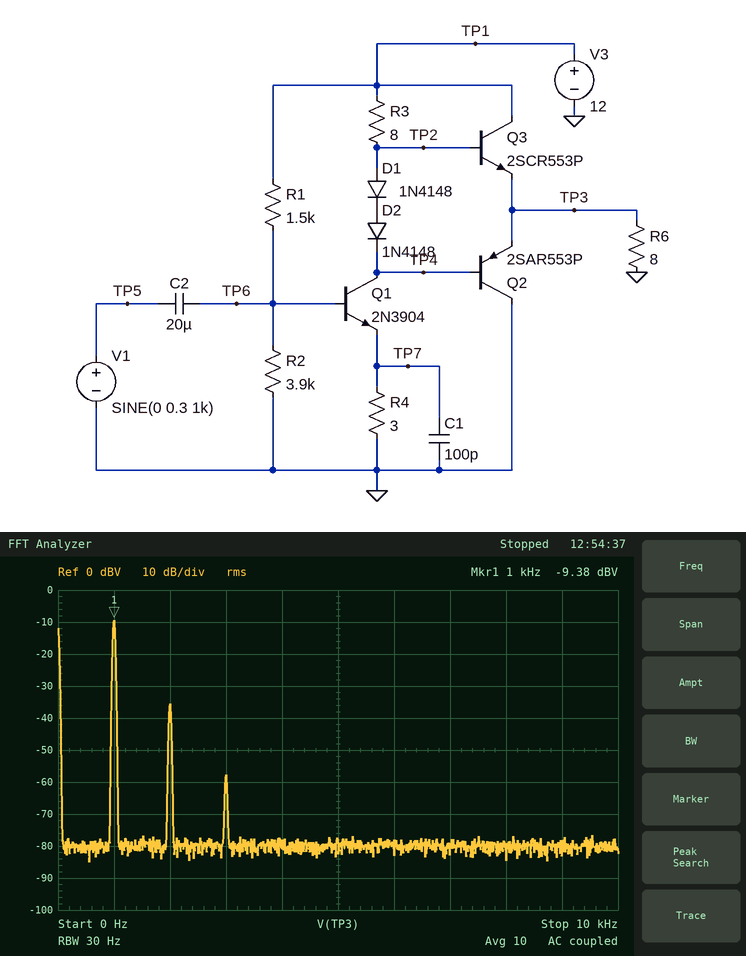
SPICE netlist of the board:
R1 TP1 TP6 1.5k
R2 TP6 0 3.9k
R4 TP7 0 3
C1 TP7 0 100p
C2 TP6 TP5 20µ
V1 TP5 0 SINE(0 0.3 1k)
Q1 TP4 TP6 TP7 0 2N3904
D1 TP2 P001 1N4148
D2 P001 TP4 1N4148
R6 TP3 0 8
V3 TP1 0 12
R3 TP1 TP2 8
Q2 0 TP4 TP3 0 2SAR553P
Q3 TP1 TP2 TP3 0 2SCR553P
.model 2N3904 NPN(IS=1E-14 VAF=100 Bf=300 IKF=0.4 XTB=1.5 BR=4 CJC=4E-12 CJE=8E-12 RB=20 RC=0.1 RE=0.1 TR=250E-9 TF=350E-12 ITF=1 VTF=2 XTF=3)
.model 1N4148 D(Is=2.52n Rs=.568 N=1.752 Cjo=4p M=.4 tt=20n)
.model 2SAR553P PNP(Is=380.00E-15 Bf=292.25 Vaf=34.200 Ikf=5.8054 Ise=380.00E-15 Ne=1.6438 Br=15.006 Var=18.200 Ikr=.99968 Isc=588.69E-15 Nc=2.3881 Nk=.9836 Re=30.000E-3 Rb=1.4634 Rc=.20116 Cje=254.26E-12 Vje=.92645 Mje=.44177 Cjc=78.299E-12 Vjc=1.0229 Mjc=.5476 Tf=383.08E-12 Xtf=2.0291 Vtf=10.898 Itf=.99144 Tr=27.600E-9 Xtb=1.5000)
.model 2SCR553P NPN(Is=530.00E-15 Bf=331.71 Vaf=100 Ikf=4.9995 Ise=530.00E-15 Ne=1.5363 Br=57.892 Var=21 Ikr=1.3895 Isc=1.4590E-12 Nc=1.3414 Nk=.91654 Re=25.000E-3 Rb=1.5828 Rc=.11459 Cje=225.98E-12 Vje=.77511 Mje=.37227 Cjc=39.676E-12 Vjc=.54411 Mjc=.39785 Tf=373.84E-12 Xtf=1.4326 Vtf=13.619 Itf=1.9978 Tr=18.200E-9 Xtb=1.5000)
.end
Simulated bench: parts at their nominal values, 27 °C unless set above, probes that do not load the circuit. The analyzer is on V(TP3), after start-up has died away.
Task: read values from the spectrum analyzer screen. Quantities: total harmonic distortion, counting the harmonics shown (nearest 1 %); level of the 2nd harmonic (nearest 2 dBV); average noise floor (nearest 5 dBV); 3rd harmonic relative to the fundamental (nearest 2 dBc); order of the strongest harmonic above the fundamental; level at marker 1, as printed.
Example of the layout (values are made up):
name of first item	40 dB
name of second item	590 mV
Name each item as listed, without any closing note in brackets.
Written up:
total harmonic distortion, counting the harmonics shown	5 %
level of the 2nd harmonic	-36 dBV
average noise floor	-80 dBV
3rd harmonic relative to the fundamental	-48 dBc
order of the strongest harmonic above the fundamental	2
level at marker 1, as printed	-9.38 dBV
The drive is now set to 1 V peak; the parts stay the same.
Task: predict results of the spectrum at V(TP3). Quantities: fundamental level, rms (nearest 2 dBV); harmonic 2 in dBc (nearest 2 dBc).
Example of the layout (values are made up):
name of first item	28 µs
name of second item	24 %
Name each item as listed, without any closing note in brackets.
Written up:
fundamental level, rms	2 dBV
harmonic 2 in dBc	-14 dBc
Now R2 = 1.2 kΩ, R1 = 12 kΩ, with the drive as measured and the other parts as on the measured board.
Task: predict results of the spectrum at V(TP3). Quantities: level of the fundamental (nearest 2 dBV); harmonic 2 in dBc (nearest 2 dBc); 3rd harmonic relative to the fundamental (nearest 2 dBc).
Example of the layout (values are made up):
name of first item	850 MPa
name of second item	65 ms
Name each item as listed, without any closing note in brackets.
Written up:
level of the fundamental	-6 dBV
harmonic 2 in dBc	-14 dBc
3rd harmonic relative to the fundamental	-26 dBc
